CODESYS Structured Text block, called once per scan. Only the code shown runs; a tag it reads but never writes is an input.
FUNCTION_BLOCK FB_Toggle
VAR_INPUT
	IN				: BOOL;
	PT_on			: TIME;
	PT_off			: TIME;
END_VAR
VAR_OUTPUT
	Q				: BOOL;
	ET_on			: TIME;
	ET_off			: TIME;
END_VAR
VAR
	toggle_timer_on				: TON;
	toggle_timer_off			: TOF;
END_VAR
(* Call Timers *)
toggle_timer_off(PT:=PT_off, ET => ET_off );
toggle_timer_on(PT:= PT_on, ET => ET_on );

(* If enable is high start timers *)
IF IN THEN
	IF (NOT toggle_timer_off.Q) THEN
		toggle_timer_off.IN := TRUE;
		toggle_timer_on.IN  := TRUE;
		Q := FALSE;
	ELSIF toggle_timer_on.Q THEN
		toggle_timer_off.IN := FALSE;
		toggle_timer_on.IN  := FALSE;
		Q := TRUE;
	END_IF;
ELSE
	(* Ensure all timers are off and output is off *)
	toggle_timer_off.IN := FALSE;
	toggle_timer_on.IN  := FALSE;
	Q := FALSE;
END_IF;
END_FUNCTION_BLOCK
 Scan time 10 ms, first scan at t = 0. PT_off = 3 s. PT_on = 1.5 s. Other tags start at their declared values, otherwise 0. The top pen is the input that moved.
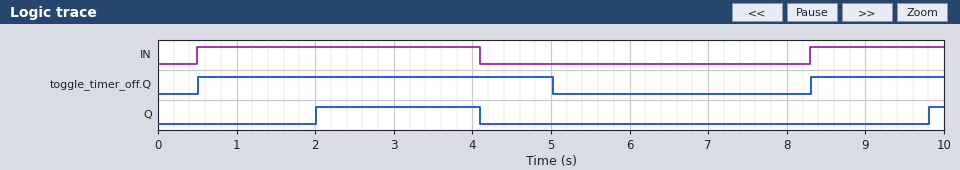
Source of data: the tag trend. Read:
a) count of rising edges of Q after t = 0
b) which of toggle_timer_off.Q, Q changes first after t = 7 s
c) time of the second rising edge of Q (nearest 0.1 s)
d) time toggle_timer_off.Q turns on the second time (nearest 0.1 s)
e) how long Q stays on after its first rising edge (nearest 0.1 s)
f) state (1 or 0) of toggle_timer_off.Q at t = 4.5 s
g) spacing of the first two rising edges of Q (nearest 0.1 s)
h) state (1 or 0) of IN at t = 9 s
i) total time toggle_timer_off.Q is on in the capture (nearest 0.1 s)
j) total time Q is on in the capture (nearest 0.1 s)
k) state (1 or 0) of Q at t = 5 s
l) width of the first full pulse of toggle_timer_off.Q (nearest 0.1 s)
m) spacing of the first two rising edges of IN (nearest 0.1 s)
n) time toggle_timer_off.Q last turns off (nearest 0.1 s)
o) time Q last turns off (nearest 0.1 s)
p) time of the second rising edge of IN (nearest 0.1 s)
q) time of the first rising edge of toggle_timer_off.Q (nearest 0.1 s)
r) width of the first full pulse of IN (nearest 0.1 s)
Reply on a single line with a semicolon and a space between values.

2; toggle_timer_off.Q; 9.8 s; 8.3 s; 2.1 s; 1; 7.8 s; 1; 6.2 s; 2.3 s; 0; 4.5 s; 7.8 s; 5.0 s; 4.1 s; 8.3 s; 0.5 s; 3.6 s
